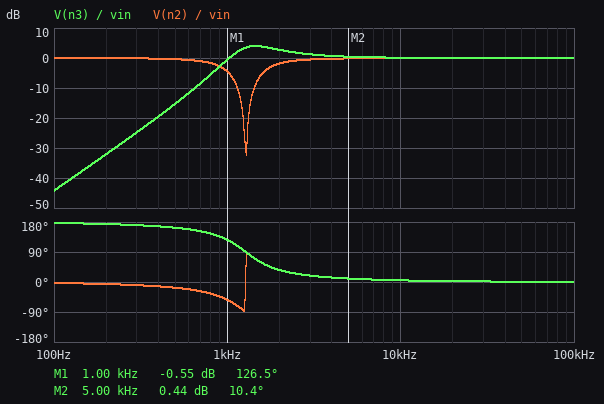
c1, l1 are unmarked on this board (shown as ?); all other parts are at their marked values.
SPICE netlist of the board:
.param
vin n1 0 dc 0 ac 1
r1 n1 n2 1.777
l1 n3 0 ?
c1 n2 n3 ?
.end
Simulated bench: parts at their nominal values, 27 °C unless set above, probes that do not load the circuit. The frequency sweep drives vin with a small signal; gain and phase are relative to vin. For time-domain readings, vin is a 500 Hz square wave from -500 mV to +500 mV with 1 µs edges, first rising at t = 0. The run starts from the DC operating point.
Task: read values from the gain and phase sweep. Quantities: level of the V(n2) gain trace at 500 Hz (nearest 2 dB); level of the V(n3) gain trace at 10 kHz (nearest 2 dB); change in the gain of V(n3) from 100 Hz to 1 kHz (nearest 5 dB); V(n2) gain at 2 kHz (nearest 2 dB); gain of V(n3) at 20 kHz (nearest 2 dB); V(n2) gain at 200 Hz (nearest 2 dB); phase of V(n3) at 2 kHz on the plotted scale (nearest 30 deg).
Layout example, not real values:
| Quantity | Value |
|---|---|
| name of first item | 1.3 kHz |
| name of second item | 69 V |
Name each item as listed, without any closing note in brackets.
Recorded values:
| Quantity | Value |
|---|---|
| level of the V(n2) gain trace at 500 Hz | 0 dB |
| level of the V(n3) gain trace at 10 kHz | 0 dB |
| change in the gain of V(n3) from 100 Hz to 1 kHz | 45 dB |
| V(n2) gain at 2 kHz | -2 dB |
| gain of V(n3) at 20 kHz | 0 dB |
| V(n2) gain at 200 Hz | 0 dB |
| phase of V(n3) at 2 kHz on the plotted scale | 30 deg |
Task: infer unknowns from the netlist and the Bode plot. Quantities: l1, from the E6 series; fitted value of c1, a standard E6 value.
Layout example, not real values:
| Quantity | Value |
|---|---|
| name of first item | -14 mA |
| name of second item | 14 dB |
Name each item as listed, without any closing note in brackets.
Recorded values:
| Quantity | Value |
|---|---|
| l1, from the E6 series | 330 µH |
| fitted value of c1, a standard E6 value | 47 µF |
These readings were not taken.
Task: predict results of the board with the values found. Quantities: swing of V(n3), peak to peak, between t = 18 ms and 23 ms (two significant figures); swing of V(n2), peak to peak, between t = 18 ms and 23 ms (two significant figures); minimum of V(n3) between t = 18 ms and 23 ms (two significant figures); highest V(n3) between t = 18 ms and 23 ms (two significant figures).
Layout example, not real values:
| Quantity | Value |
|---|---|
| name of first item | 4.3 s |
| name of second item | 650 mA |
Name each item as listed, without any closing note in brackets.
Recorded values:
| Quantity | Value |
|---|---|
| swing of V(n3), peak to peak, between t = 18 ms and 23 ms | 2.0 V |
| swing of V(n2), peak to peak, between t = 18 ms and 23 ms | 1.3 V |
| minimum of V(n3) between t = 18 ms and 23 ms | -1.0 V |
| highest V(n3) between t = 18 ms and 23 ms | 1.0 V |
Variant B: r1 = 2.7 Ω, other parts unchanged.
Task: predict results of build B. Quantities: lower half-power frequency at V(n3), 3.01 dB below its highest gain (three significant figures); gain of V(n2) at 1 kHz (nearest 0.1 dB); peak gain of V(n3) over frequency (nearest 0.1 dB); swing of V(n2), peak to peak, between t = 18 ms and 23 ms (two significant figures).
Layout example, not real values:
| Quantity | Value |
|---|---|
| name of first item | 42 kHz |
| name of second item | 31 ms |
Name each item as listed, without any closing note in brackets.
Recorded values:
| Quantity | Value |
|---|---|
| lower half-power frequency at V(n3), 3.01 dB below its highest gain | 1.10 kHz |
| gain of V(n2) at 1 kHz | -7.2 dB |
| peak gain of V(n3) over frequency | 1.1 dB |
| swing of V(n2), peak to peak, between t = 18 ms and 23 ms | 1.2 V |
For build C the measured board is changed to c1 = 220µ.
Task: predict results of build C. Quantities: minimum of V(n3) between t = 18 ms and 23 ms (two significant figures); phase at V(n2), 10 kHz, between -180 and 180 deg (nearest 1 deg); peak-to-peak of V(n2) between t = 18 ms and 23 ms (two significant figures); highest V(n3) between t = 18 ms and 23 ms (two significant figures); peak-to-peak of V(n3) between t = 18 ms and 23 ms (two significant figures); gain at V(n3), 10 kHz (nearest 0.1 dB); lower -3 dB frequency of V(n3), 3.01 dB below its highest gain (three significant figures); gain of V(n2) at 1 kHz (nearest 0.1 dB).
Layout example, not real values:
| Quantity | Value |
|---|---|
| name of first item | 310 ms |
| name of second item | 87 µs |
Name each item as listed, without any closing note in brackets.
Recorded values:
| Quantity | Value |
|---|---|
| minimum of V(n3) between t = 18 ms and 23 ms | -1.1 V |
| phase at V(n2), 10 kHz, between -180 and 180 deg | 5 deg |
| peak-to-peak of V(n2) between t = 18 ms and 23 ms | 1.2 V |
| highest V(n3) between t = 18 ms and 23 ms | 1.1 V |
| peak-to-peak of V(n3) between t = 18 ms and 23 ms | 2.2 V |
| gain at V(n3), 10 kHz | 0 dB |
| lower -3 dB frequency of V(n3), 3.01 dB below its highest gain | 606 Hz |
| gain of V(n2) at 1 kHz | -4.4 dB |
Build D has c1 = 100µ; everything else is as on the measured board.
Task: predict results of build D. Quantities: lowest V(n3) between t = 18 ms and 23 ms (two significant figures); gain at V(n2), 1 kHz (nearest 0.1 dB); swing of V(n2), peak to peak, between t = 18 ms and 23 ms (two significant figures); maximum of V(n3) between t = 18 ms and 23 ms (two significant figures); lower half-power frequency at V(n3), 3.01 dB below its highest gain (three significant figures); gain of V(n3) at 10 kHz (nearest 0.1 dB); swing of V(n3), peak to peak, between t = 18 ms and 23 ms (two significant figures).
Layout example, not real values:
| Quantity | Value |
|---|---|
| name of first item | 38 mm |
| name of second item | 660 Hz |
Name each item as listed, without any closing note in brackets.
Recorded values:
| Quantity | Value |
|---|---|
| lowest V(n3) between t = 18 ms and 23 ms | -950 mV |
| gain at V(n2), 1 kHz | -11.6 dB |
| swing of V(n2), peak to peak, between t = 18 ms and 23 ms | 1.2 V |
| maximum of V(n3) between t = 18 ms and 23 ms | 950 mV |
| lower half-power frequency at V(n3), 3.01 dB below its highest gain | 747 Hz |
| gain of V(n3) at 10 kHz | 0 dB |
| swing of V(n3), peak to peak, between t = 18 ms and 23 ms | 1.9 V |
